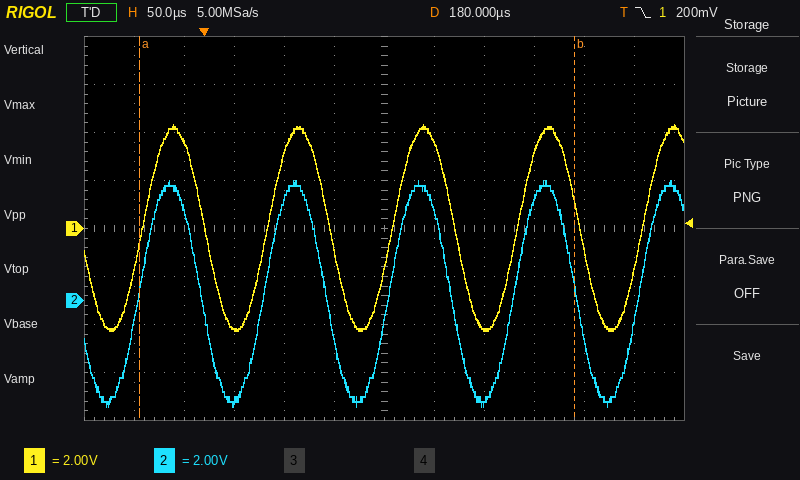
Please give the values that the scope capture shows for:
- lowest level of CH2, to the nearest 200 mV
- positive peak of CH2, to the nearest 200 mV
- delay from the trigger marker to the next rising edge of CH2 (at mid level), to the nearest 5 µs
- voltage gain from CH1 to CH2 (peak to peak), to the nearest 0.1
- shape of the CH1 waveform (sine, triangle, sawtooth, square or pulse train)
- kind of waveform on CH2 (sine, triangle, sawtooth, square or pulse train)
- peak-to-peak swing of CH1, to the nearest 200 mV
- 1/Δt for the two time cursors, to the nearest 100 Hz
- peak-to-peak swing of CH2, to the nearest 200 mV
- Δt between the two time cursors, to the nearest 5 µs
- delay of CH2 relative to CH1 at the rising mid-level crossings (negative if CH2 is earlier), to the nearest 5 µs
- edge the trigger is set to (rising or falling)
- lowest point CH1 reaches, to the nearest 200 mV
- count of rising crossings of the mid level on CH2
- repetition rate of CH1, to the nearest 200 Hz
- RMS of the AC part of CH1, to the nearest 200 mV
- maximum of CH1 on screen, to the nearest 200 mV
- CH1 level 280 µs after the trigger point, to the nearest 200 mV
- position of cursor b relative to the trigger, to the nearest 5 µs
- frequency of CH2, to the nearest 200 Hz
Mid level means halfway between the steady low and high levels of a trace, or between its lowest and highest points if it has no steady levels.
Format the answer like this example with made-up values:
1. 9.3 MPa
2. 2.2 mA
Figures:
1. -4.4 V
2. 5.0 V
3. 60 µs
4. 1.1
5. sine
6. sine
7. 8.6 V
8. 2.3 kHz
9. 9.4 V
10. 435 µs
11. -5 µs
12. falling
13. -4.2 V
14. 5
15. 8.0 kHz
16. 3.0 V
17. 4.4 V
18. -4.2 V
19. +370 µs
20. 8.0 kHz
